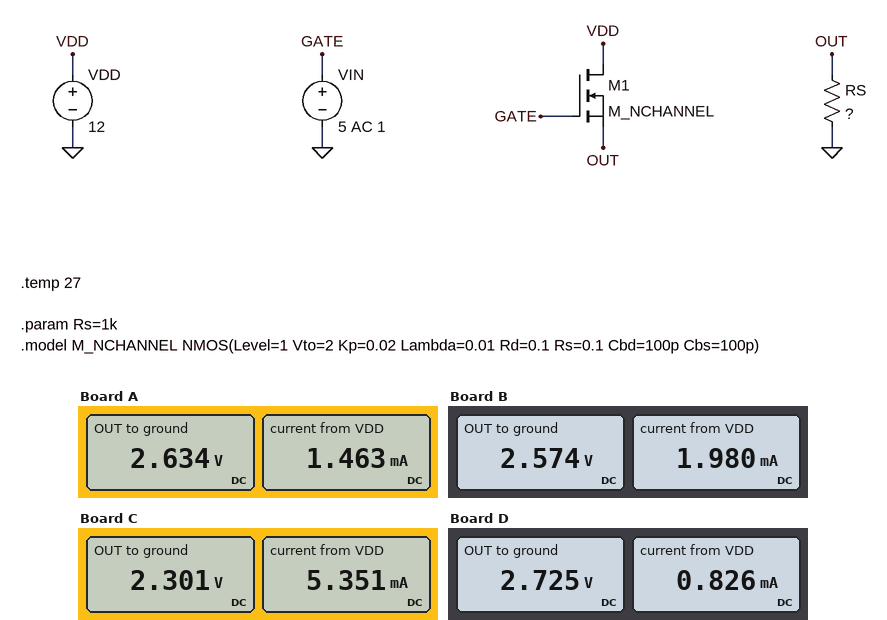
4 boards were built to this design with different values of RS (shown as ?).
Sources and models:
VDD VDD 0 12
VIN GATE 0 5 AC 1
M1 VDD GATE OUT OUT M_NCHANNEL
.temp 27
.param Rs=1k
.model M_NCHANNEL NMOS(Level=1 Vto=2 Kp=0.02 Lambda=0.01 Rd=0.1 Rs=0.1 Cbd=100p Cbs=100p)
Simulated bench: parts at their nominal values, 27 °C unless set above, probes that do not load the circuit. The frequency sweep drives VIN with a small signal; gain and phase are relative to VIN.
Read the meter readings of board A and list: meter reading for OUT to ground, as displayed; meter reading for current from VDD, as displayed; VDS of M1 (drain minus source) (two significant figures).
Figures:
2.634 V
1.463 mA
9.4 V
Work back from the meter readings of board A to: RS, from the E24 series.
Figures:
1.8 kΩ
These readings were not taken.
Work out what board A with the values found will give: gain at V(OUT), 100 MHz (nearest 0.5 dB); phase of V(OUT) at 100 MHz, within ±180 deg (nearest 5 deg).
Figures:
-8.0 dB
-65 deg
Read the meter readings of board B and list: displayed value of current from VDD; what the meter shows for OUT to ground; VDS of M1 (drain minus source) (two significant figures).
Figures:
1.980 mA
2.574 V
9.4 V
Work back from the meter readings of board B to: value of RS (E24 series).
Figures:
1.3 kΩ
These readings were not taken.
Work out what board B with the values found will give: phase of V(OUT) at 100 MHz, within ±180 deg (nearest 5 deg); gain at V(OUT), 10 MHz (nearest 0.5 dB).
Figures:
-60 deg
-1.0 dB
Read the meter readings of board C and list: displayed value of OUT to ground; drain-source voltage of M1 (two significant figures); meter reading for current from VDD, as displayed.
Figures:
2.301 V
9.7 V
5.351 mA
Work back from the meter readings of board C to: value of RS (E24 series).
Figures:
430 Ω
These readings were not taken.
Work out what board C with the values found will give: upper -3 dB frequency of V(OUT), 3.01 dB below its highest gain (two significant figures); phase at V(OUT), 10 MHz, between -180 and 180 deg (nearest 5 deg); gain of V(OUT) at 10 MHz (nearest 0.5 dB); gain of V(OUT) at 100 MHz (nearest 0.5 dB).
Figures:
100 MHz
-5 deg
-1.5 dB
-4.0 dB
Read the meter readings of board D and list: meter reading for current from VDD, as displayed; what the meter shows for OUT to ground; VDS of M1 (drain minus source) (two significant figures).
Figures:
0.826 mA
2.725 V
9.3 V
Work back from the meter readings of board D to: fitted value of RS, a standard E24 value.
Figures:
3.3 kΩ
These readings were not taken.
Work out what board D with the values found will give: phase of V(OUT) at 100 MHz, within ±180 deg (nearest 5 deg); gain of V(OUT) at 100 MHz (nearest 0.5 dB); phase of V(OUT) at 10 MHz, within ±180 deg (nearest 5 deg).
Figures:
-70 deg
-10.0 dB
-15 deg
